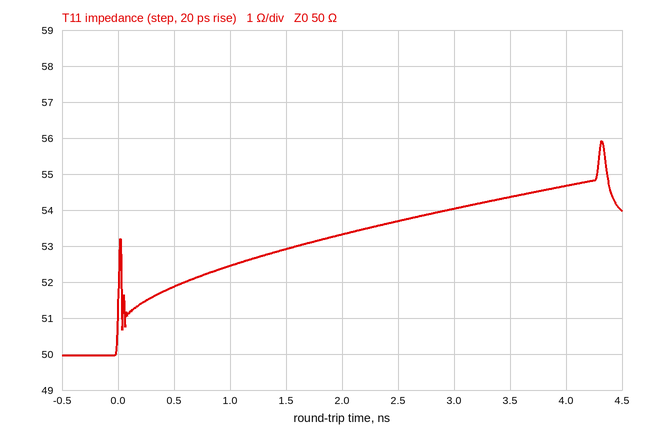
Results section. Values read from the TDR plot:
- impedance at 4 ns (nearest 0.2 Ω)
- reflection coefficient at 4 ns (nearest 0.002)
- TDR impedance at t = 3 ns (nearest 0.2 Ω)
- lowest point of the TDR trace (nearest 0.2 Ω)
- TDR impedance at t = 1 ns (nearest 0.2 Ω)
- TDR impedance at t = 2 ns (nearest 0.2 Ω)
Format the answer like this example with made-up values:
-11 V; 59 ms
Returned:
54.6 Ω; +0.044; 54.0 Ω; 50.0 Ω; 52.4 Ω; 53.4 Ω
